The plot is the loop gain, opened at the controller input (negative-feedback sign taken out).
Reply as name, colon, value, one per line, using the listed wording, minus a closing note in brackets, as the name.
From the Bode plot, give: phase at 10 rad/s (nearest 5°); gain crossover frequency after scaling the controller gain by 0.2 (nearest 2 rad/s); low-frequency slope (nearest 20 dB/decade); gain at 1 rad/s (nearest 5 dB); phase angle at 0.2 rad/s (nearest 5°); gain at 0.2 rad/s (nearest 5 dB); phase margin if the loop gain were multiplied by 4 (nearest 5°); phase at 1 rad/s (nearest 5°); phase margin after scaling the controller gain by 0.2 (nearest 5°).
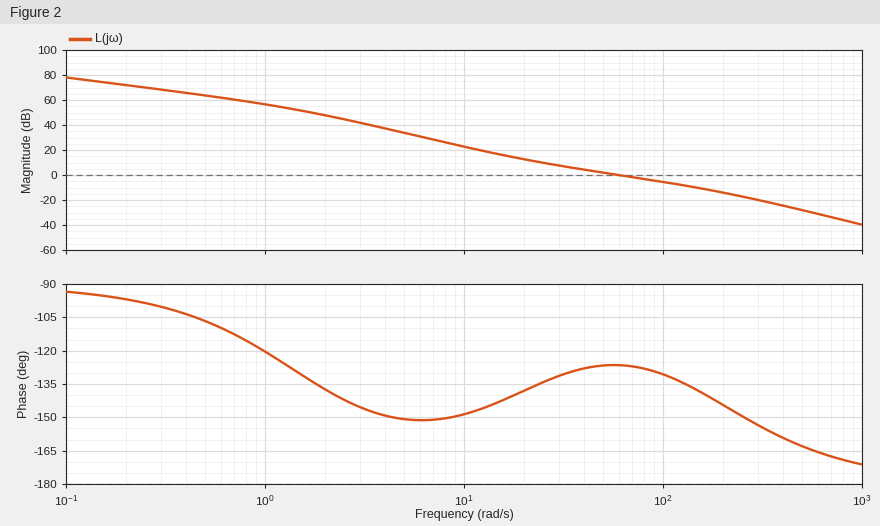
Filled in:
phase at 10 rad/s: -150°
gain crossover frequency after scaling the controller gain by 0.2: 18 rad/s
low-frequency slope: -20 dB/decade
gain at 1 rad/s: 55 dB
phase angle at 0.2 rad/s: -95°
gain at 0.2 rad/s: 70 dB
phase margin if the loop gain were multiplied by 4: 40°
phase at 1 rad/s: -120°
phase margin after scaling the controller gain by 0.2: 40°
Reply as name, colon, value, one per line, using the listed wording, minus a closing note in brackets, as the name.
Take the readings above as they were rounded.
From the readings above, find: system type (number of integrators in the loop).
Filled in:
system type: 1
